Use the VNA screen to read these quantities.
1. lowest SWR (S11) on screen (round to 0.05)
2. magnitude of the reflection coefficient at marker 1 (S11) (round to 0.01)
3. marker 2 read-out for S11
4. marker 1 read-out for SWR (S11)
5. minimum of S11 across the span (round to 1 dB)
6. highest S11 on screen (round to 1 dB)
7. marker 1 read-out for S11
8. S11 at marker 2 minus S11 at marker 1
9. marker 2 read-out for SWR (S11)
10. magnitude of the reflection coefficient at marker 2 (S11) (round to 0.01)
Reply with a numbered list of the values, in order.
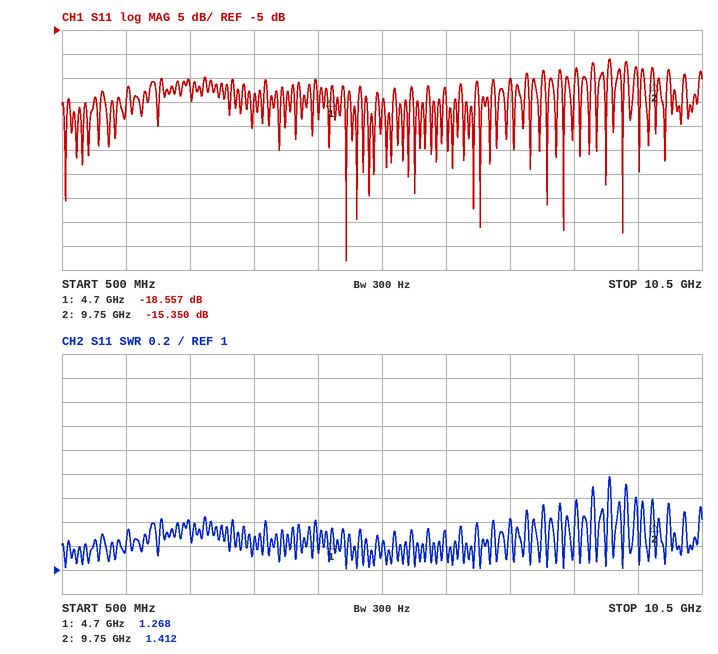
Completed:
1. 1.00
2. 0.12
3. -15.350 dB
4. 1.268
5. -53 dB
6. -11 dB
7. -18.557 dB
8. 3.207 dB
9. 1.412
10. 0.17
